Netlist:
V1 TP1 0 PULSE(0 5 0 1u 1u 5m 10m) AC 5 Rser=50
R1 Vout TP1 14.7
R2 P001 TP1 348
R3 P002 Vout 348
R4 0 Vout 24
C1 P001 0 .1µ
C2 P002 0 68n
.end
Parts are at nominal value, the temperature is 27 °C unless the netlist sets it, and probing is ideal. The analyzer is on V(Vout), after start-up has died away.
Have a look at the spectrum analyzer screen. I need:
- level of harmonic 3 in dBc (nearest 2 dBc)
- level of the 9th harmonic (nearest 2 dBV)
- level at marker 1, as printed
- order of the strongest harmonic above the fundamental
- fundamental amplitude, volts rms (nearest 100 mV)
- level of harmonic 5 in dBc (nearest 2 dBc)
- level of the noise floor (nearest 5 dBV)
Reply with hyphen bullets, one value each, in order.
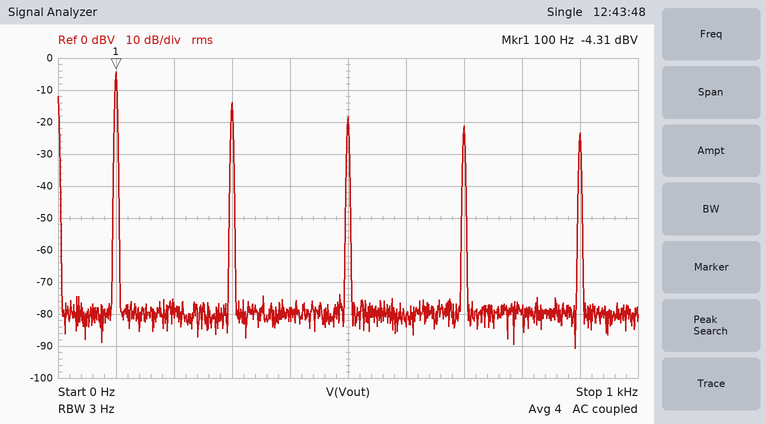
- -10 dBc
- -24 dBV
- -4.31 dBV
- 3
- 600 mV
- -14 dBc
- -80 dBV
